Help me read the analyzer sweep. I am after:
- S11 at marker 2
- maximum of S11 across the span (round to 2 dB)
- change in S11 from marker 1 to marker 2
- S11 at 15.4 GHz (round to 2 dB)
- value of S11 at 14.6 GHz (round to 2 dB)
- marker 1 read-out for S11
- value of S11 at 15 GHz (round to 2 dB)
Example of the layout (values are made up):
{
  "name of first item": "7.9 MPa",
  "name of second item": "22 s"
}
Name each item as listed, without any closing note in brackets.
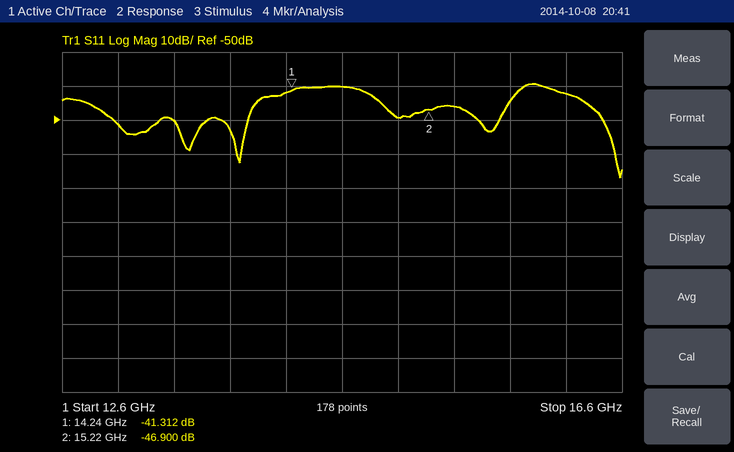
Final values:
{
  "S11 at marker 2": "-46.900 dB",
  "maximum of S11 across the span": "-40 dB",
  "change in S11 from marker 1 to marker 2": "-5.588 dB",
  "S11 at 15.4 GHz": "-46 dB",
  "value of S11 at 14.6 GHz": "-40 dB",
  "marker 1 read-out for S11": "-41.312 dB",
  "value of S11 at 15 GHz": "-50 dB"
}
